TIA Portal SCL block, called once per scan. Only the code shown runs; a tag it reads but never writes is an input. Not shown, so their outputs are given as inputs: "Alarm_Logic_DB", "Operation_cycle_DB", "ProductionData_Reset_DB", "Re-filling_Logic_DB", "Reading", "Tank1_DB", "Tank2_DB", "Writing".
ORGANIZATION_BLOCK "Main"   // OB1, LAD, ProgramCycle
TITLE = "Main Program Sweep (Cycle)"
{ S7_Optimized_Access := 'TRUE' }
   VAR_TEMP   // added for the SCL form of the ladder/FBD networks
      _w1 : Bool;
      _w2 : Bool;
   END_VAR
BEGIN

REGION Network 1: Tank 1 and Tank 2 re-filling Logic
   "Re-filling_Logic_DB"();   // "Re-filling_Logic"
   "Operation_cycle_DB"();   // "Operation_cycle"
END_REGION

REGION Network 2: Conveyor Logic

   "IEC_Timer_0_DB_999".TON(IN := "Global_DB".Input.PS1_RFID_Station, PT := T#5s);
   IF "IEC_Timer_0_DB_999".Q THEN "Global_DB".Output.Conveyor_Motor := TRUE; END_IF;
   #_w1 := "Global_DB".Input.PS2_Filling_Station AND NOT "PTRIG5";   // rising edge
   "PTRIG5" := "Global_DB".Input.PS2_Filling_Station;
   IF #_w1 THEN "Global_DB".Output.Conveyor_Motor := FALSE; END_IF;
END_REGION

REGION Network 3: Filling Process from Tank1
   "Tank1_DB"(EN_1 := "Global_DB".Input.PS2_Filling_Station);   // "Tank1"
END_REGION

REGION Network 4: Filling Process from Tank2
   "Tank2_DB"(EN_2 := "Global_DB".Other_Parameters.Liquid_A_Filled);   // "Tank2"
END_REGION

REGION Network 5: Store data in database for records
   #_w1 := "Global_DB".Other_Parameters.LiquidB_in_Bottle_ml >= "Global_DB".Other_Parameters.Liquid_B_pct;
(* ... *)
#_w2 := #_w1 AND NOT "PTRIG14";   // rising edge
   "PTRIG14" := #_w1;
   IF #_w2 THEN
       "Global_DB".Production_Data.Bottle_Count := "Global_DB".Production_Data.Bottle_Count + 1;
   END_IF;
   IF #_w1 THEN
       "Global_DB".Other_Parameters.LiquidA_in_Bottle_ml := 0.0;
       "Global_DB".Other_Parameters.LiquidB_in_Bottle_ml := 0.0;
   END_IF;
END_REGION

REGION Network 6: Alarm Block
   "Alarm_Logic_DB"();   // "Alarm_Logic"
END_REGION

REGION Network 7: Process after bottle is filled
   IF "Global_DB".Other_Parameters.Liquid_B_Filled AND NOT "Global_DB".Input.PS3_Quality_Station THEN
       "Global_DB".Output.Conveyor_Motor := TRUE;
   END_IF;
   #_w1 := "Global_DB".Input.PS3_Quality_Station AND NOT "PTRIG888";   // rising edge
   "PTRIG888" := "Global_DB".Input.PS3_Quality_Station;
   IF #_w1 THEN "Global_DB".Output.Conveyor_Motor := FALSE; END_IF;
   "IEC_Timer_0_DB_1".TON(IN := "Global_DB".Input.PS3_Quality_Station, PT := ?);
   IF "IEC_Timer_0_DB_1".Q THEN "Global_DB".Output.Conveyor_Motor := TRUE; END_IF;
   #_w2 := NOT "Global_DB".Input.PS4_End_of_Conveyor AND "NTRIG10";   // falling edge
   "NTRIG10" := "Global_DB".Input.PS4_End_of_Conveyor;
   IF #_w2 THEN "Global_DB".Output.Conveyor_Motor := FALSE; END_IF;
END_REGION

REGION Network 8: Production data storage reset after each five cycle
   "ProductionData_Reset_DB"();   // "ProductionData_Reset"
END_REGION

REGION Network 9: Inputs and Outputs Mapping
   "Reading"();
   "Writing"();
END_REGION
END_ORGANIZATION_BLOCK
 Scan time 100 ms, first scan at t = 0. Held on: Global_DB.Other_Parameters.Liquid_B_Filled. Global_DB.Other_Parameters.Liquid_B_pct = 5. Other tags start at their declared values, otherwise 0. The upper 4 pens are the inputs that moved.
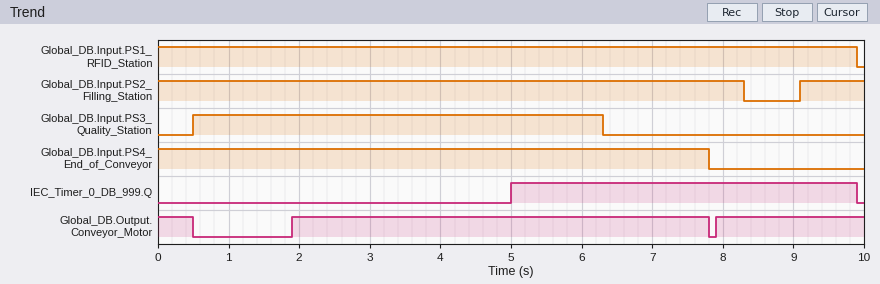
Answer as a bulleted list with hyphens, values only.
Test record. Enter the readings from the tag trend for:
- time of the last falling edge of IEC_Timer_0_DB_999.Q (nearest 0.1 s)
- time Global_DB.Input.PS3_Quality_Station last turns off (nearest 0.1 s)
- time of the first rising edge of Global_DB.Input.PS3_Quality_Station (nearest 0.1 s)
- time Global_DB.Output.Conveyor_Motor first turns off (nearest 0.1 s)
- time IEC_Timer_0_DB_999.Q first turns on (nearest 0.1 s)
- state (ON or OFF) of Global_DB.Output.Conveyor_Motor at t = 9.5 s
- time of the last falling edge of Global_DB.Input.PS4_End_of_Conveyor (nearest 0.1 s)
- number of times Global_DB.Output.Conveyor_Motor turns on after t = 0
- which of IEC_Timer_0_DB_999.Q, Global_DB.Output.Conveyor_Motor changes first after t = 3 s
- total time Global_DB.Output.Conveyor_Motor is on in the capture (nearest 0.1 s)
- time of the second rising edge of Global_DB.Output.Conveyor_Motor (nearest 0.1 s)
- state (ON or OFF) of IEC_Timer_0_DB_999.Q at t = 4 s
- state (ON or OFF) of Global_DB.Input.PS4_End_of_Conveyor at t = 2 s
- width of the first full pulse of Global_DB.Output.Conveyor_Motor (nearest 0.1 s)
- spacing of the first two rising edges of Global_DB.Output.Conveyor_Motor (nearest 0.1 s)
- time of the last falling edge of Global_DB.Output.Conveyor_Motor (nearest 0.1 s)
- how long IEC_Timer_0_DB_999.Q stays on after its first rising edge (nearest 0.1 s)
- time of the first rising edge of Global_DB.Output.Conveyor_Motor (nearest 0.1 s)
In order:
- 9.9 s
- 6.3 s
- 0.5 s
- 0.5 s
- 5.0 s
- ON
- 7.8 s
- 2
- IEC_Timer_0_DB_999.Q
- 8.5 s
- 7.9 s
- OFF
- ON
- 5.9 s
- 6.0 s
- 7.8 s
- 4.9 s
- 1.9 s
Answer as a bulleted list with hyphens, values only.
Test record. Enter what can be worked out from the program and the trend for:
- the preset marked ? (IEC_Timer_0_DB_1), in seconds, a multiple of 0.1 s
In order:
- 1.4 s
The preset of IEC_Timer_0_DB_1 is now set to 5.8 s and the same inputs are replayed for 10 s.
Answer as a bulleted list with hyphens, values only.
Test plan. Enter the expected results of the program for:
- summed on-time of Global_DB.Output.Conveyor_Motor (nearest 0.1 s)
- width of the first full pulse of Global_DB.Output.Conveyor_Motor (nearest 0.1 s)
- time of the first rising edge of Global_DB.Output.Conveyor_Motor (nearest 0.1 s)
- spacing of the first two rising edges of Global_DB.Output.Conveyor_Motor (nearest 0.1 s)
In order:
- 5.4 s
- 2.8 s
- 5.0 s
- 2.9 s
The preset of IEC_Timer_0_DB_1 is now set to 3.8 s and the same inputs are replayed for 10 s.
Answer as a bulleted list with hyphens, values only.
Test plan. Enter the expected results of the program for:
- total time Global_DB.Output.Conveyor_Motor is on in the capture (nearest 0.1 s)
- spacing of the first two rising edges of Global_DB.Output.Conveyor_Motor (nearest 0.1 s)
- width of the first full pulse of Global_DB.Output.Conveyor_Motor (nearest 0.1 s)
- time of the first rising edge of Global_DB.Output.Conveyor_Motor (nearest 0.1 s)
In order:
- 6.1 s
- 3.6 s
- 3.5 s
- 4.3 s
